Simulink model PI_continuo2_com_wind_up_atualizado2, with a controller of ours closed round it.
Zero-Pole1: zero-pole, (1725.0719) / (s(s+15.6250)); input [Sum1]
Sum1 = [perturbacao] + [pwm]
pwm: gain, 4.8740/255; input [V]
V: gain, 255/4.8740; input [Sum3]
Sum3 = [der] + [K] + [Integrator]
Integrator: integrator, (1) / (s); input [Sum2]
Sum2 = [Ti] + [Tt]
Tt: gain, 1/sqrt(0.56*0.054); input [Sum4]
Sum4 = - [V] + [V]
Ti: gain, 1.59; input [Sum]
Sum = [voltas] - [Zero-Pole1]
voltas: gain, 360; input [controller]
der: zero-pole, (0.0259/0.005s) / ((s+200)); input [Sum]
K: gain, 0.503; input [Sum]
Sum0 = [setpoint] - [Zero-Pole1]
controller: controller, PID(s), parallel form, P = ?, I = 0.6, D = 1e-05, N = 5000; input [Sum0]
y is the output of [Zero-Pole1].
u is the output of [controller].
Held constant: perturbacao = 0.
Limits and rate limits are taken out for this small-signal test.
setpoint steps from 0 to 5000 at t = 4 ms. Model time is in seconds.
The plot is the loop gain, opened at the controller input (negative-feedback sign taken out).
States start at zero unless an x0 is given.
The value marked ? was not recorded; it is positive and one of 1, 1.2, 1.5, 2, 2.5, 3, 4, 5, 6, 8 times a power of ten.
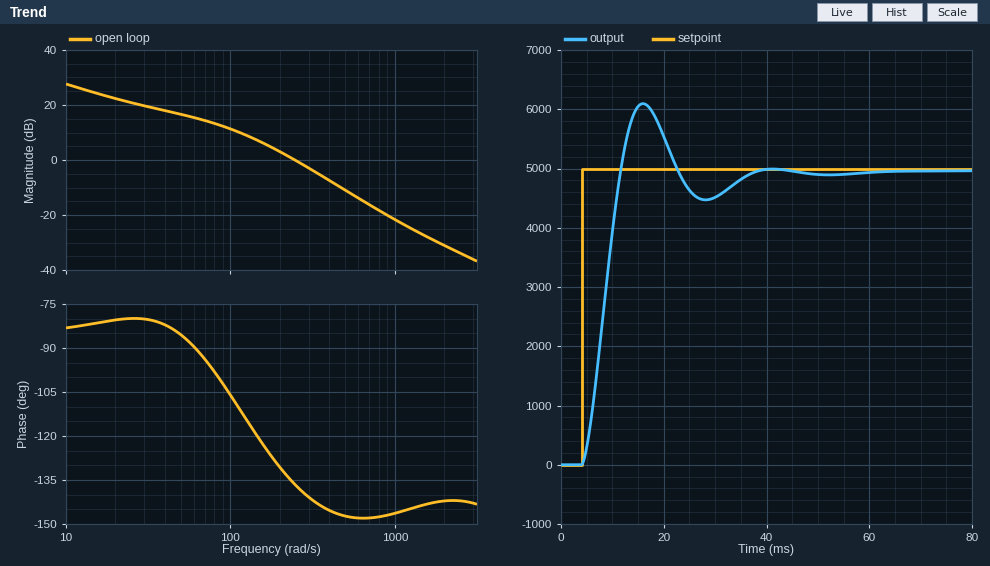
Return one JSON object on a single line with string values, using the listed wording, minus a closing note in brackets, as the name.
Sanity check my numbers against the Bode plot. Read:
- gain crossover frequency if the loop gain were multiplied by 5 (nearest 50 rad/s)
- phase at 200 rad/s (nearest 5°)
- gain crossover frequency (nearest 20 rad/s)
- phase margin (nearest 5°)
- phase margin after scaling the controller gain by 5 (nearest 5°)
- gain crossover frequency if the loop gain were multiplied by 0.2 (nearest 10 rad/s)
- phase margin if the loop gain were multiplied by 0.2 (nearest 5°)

{"gain crossover frequency if the loop gain were multiplied by 5": "600 rad/s", "phase at 200 rad/s": "-130°", "gain crossover frequency": "240 rad/s", "phase margin": "45°", "phase margin after scaling the controller gain by 5": "30°", "gain crossover frequency if the loop gain were multiplied by 0.2": "70 rad/s", "phase margin if the loop gain were multiplied by 0.2": "85°"}
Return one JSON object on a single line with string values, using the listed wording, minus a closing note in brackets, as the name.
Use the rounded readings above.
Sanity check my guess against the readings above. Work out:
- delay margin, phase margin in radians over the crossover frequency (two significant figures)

{"delay margin, phase margin in radians over the crossover frequency": "0.0033 s"}
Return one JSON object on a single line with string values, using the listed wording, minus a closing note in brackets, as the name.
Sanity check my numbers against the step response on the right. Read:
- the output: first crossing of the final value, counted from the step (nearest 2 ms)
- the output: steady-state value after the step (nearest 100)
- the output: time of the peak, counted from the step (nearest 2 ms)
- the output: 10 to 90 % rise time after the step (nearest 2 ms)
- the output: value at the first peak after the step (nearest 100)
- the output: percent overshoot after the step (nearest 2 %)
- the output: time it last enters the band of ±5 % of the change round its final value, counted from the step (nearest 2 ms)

{"the output: first crossing of the final value, counted from the step": "8 ms", "the output: steady-state value after the step": "5000", "the output: time of the peak, counted from the step": "12 ms", "the output: 10 to 90 % rise time after the step": "6 ms", "the output: value at the first peak after the step": "6100", "the output: percent overshoot after the step": "22 %", "the output: time it last enters the band of ±5 % of the change round its final value, counted from the step": "30 ms"}
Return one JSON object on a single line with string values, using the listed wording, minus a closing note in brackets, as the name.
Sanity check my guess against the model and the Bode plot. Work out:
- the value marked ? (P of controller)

{"the value marked ?": "0.02"}
